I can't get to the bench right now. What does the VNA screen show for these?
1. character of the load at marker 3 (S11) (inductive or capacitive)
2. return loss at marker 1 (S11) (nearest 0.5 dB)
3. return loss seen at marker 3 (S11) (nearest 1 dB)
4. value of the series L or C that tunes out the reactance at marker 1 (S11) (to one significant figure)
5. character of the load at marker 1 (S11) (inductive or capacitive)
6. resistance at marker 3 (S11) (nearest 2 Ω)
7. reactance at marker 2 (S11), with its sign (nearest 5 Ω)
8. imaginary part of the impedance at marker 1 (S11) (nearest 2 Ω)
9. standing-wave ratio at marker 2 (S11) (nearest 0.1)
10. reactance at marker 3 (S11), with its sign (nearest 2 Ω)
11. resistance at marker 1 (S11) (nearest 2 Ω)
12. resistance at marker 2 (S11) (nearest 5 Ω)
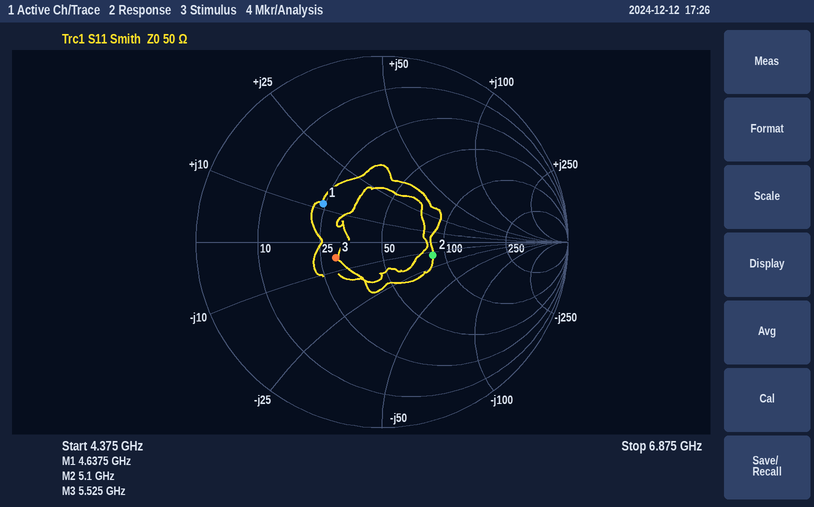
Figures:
capacitive
8.5 dB
12 dB
3 pF
inductive
30 Ω
-15 Ω
+12 Ω
1.8
-6 Ω
24 Ω
85 Ω
